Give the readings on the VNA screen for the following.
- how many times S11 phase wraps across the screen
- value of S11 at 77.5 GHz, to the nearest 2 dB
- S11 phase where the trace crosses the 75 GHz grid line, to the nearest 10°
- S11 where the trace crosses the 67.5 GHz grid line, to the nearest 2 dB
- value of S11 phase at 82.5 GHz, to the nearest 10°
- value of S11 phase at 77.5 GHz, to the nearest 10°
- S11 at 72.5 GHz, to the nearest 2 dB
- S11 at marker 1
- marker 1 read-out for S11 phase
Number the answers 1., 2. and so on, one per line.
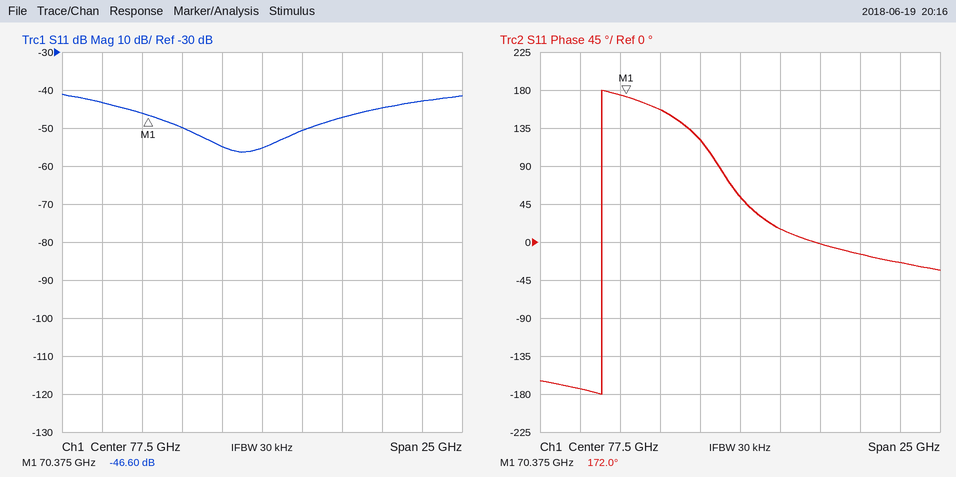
1. 1
2. -56 dB
3. 120°
4. -44 dB
5. 0°
6. 50°
7. -50 dB
8. -46.60 dB
9. 172.0°
